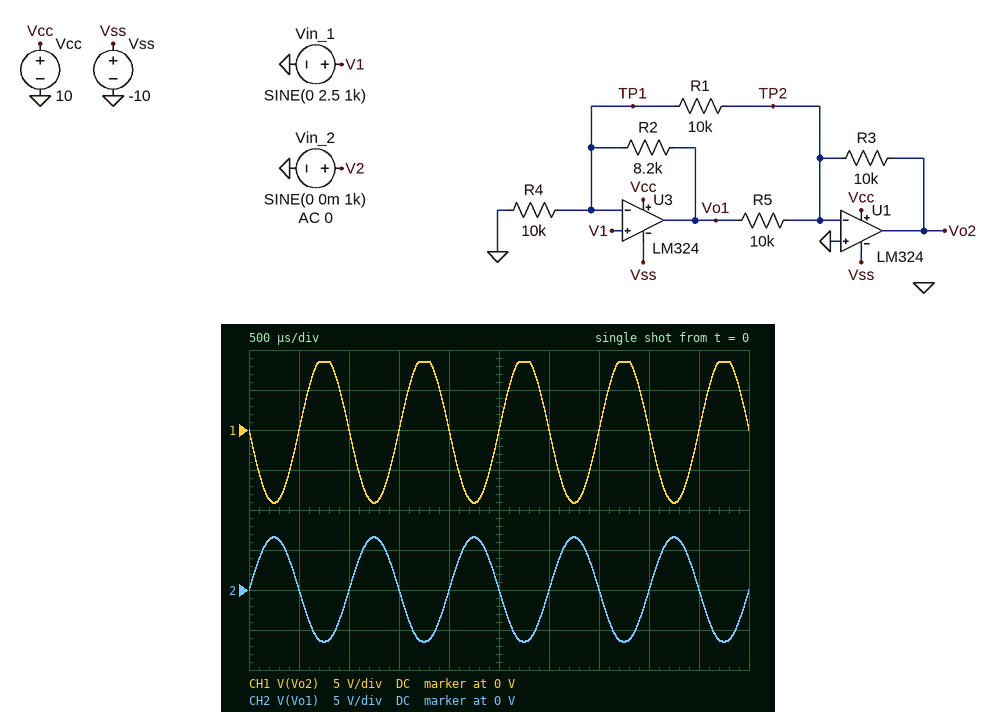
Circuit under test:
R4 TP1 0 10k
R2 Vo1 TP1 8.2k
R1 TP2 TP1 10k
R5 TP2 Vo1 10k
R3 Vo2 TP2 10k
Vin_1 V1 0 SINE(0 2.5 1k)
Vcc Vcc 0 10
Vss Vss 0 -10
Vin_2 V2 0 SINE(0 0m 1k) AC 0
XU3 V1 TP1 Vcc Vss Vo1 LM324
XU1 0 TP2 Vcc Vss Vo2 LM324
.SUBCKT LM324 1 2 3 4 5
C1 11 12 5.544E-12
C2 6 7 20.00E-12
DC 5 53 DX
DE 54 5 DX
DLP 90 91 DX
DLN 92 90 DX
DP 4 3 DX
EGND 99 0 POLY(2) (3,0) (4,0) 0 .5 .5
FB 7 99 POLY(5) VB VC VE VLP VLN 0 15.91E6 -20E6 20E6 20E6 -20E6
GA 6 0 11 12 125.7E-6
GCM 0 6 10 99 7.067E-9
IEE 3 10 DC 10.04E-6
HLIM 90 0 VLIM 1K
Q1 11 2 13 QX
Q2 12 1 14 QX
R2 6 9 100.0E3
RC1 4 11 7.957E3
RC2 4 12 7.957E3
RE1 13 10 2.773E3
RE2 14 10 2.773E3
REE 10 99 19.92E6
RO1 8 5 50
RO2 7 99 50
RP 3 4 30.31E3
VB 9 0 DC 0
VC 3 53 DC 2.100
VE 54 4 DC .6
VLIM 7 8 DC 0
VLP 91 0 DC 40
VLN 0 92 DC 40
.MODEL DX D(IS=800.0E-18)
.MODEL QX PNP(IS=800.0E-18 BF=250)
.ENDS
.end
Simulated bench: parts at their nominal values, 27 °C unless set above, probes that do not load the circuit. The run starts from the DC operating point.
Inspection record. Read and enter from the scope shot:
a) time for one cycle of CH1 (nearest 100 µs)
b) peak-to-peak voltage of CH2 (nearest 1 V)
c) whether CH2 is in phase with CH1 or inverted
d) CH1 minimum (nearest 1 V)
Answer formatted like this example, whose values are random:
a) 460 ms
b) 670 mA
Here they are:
a) 1.0 ms
b) 13 V
c) inverted
d) -9 V
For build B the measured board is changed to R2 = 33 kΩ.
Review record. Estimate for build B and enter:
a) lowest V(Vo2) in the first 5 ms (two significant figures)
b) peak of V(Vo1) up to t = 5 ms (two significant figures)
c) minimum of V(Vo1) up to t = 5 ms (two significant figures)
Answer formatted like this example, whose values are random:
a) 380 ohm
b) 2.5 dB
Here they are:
a) -9.6 V
b) 8.5 V
c) -10 V
